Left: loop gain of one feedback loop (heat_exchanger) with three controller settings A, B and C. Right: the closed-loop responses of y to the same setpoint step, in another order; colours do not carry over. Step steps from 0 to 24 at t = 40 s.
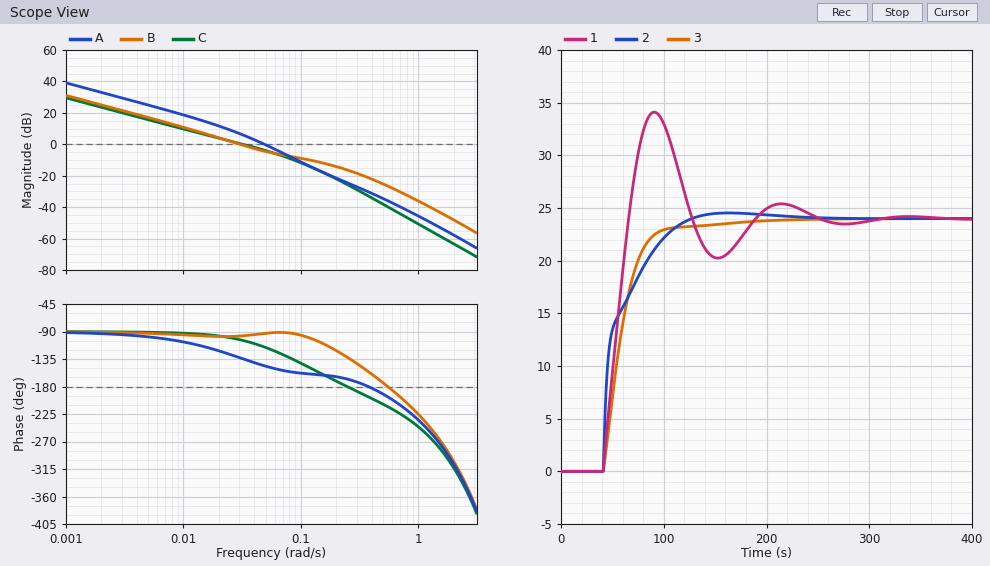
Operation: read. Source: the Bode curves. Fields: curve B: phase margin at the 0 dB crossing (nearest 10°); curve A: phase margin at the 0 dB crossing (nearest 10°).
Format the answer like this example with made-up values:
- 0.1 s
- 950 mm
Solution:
- 80°
- 30°
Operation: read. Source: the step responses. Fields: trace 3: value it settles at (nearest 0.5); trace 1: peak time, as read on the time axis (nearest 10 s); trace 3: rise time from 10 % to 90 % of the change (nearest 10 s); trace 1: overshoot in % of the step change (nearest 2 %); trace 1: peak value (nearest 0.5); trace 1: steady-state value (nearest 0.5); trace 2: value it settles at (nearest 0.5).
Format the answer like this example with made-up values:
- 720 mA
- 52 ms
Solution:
- 24.0
- 90 s
- 40 s
- 42 %
- 34.0
- 24.0
- 24.0
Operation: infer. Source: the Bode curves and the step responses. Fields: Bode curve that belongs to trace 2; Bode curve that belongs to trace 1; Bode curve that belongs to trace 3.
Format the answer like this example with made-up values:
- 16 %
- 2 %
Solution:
- B
- A
- C
